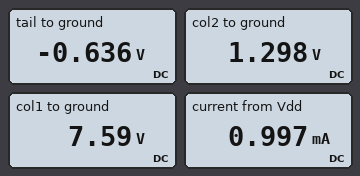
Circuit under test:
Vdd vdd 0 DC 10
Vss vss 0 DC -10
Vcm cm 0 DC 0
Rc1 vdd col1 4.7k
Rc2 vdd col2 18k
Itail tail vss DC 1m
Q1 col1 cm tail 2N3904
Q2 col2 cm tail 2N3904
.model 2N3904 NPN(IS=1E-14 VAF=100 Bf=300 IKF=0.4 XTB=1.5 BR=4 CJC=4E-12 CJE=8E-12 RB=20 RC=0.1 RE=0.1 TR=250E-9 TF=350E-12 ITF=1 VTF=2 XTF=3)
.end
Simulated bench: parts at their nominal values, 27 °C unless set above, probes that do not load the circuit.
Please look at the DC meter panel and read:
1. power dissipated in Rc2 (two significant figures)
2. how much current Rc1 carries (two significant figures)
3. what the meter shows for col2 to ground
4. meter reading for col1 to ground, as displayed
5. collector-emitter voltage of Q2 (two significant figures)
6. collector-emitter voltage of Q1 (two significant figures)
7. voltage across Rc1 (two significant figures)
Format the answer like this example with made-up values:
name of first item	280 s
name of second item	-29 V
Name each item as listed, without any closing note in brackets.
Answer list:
power dissipated in Rc2	4.2 mW
how much current Rc1 carries	510 µA
what the meter shows for col2 to ground	1.298 V
meter reading for col1 to ground, as displayed	7.59 V
collector-emitter voltage of Q2	1.9 V
collector-emitter voltage of Q1	8.2 V
voltage across Rc1	2.4 V
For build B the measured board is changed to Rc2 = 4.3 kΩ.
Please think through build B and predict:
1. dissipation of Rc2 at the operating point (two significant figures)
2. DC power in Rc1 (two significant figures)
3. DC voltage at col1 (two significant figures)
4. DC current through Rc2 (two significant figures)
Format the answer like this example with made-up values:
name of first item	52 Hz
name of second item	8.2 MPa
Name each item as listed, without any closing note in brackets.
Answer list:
dissipation of Rc2 at the operating point	1.1 mW
DC power in Rc1	1.2 mW
DC voltage at col1	7.7 V
DC current through Rc2	500 µA
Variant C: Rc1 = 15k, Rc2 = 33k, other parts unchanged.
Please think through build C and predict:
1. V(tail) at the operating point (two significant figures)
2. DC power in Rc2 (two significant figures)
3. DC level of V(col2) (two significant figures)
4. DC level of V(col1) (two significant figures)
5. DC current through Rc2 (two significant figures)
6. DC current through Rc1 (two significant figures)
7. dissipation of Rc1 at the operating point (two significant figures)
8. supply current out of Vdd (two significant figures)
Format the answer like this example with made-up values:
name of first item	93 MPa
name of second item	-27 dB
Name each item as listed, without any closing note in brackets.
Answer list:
V(tail) at the operating point	-640 mV
DC power in Rc2	3.4 mW
DC level of V(col2)	-620 mV
DC level of V(col1)	690 mV
DC current through Rc2	320 µA
DC current through Rc1	620 µA
dissipation of Rc1 at the operating point	5.8 mW
supply current out of Vdd	940 µA
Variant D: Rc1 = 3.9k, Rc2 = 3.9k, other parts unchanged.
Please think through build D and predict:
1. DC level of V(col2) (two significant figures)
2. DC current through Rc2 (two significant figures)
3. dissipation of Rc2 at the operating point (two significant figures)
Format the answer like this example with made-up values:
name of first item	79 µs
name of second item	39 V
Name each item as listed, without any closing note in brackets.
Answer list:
DC level of V(col2)	8.1 V
DC current through Rc2	500 µA
dissipation of Rc2 at the operating point	970 µW
